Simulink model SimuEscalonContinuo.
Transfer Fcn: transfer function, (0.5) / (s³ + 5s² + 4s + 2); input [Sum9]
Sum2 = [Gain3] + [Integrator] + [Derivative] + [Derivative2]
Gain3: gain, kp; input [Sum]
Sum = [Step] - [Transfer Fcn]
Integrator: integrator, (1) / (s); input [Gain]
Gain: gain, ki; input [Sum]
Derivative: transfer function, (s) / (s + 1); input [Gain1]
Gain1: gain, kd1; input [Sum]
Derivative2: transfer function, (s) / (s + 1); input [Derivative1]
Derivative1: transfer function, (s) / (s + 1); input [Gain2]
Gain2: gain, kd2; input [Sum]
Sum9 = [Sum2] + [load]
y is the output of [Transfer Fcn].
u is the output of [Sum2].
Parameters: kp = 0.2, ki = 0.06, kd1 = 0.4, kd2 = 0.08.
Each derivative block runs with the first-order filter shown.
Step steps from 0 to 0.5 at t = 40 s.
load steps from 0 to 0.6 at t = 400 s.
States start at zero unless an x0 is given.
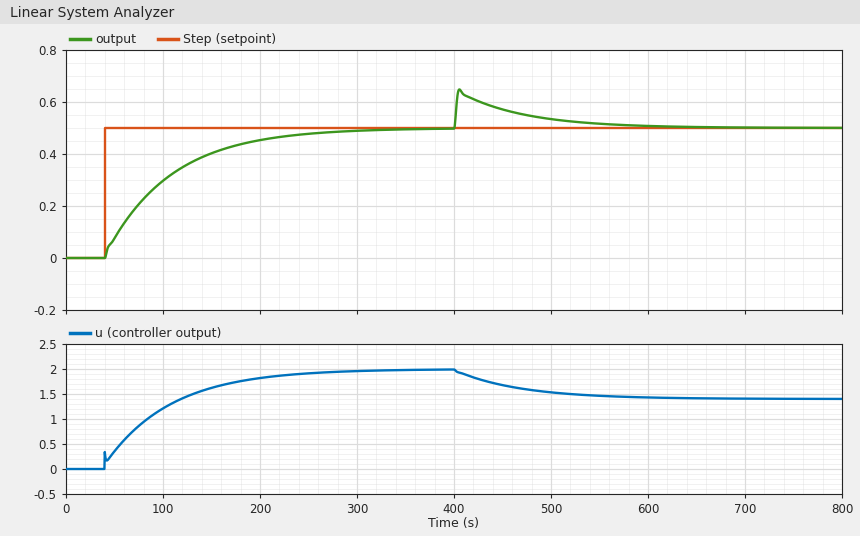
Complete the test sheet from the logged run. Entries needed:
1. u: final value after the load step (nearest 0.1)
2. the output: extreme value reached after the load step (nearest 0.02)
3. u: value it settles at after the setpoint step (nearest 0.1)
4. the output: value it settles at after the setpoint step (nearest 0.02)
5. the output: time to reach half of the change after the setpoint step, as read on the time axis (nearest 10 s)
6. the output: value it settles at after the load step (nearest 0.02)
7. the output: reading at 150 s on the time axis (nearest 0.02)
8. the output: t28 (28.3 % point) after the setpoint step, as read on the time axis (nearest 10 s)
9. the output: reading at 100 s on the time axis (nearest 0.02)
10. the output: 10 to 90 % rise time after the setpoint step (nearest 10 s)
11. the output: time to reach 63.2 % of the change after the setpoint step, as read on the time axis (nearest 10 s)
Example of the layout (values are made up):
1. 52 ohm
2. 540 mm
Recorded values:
1. 1.4
2. 0.64
3. 2.0
4. 0.50
5. 90 s
6. 0.50
7. 0.40
8. 60 s
9. 0.30
10. 150 s
11. 110 s
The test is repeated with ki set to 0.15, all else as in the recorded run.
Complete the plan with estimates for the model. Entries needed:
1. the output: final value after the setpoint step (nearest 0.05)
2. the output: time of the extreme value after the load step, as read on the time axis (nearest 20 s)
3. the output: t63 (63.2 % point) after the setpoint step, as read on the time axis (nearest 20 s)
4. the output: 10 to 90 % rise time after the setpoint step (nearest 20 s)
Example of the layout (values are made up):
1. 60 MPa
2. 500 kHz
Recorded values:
1. 0.50
2. 400 s
3. 60 s
4. 60 s
